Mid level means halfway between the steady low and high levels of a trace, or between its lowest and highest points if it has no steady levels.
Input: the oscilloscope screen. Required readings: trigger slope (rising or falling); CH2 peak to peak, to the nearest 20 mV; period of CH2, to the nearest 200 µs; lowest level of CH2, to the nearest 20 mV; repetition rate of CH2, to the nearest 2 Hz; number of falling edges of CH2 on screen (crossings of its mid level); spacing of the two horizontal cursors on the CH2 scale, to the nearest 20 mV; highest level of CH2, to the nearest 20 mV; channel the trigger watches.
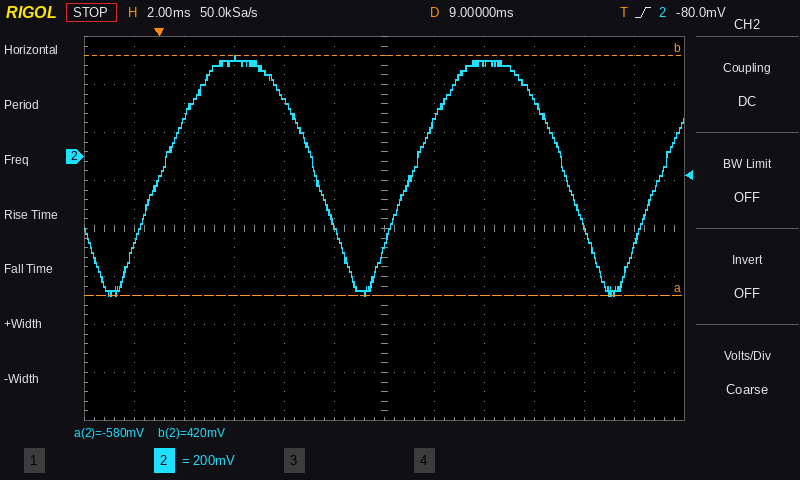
rising
1.00 V
10.0 ms
-580 mV
100 Hz
2
1.00 V
420 mV
CH2
